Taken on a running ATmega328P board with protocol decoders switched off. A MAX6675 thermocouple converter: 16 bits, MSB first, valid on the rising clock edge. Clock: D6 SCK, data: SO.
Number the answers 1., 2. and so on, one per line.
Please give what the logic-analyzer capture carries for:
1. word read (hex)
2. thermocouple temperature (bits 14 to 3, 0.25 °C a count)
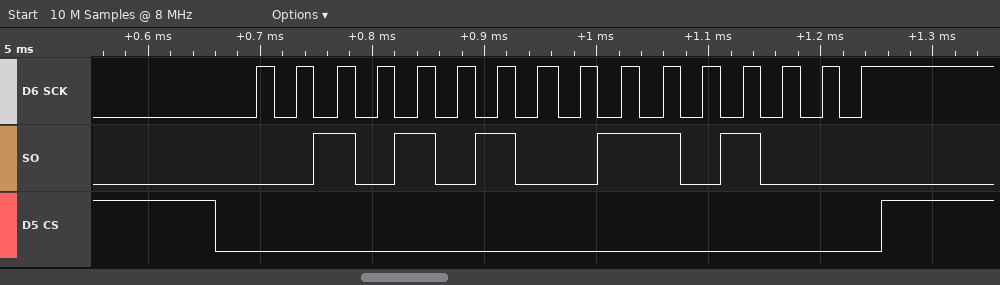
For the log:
1. 0x2A68
2. 339.25 °C
